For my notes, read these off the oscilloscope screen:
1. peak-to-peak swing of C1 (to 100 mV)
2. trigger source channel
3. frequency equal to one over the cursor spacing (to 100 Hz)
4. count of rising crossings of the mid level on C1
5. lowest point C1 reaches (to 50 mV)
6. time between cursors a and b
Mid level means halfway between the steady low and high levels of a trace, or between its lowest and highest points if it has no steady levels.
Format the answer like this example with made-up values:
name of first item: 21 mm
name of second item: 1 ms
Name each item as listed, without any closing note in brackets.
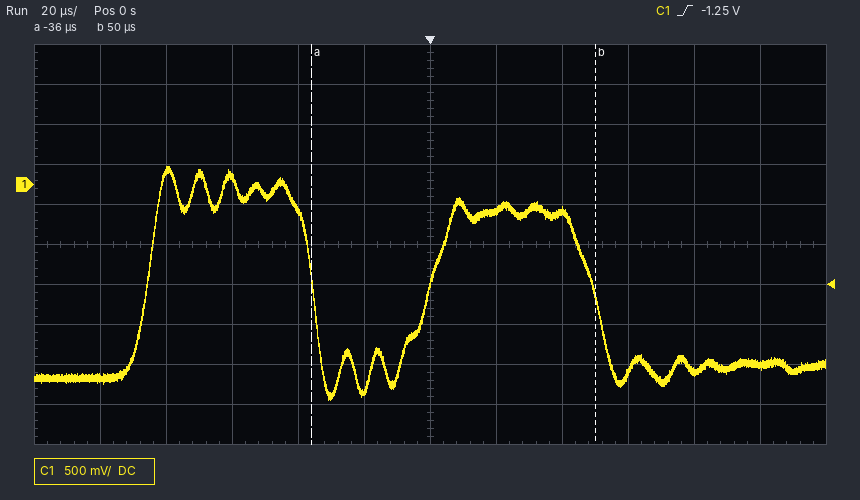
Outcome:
peak-to-peak swing of C1: 2.90 V
trigger source channel: C1
frequency equal to one over the cursor spacing: 11.6 kHz
count of rising crossings of the mid level on C1: 2
lowest point C1 reaches: -2.70 V
time between cursors a and b: 86 µs
